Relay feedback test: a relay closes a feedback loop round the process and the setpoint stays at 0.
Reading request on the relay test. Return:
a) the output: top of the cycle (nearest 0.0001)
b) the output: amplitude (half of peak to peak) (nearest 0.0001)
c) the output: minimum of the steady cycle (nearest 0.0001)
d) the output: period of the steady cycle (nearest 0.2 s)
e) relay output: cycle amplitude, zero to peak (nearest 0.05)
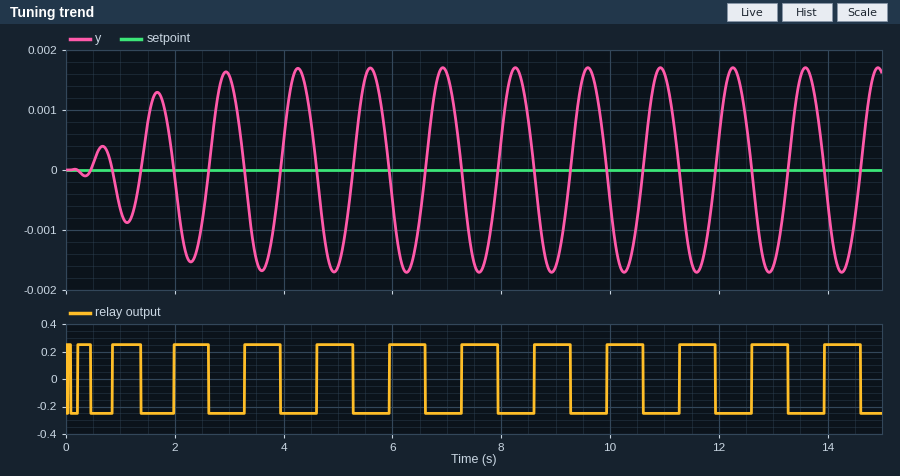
0.0017
0.0017
-0.0017
1.4 s
0.25
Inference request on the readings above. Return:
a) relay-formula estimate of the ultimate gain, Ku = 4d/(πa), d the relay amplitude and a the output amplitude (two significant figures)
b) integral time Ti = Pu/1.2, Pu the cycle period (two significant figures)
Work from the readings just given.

190
1.2 s
